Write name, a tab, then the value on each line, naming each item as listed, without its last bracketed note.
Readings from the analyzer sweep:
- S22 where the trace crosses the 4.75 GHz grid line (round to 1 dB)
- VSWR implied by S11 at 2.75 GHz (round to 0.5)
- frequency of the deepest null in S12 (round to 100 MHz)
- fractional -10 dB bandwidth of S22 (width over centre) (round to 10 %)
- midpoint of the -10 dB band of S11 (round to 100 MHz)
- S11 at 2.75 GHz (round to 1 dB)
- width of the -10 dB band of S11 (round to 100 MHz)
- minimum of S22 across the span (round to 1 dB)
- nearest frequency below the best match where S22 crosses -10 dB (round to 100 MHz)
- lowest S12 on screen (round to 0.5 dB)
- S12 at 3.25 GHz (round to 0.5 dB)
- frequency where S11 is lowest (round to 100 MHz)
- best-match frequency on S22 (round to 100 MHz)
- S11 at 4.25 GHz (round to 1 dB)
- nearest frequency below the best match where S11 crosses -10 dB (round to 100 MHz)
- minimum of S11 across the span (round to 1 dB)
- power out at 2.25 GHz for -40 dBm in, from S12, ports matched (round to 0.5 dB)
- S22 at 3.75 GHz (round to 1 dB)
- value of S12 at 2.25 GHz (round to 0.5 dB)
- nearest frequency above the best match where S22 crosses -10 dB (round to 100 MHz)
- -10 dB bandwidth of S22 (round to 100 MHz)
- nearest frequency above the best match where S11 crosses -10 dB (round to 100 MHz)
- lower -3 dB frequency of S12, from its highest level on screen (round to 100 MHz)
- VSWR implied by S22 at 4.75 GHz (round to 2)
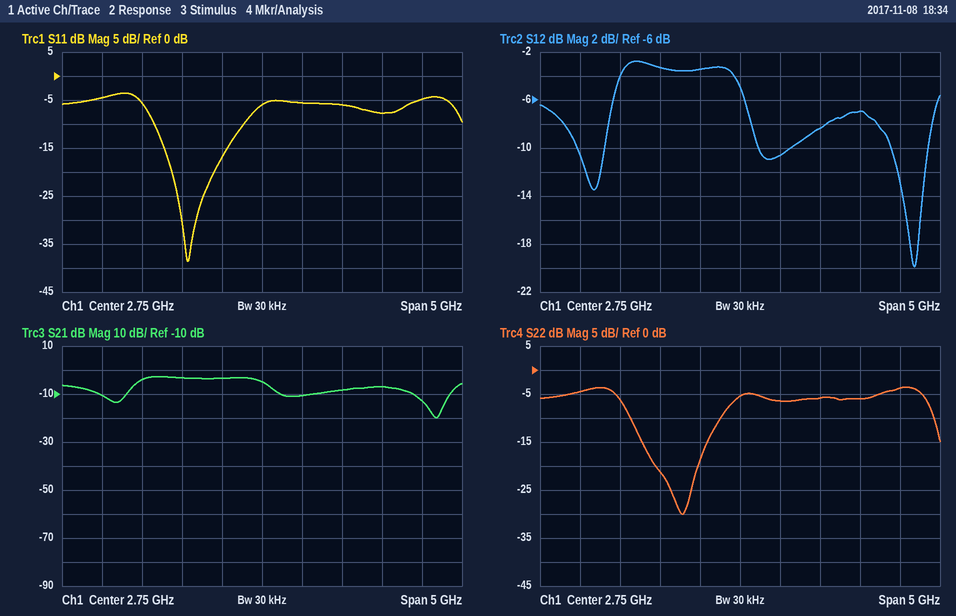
S22 where the trace crosses the 4.75 GHz grid line	-4 dB
VSWR implied by S11 at 2.75 GHz	3.0
frequency of the deepest null in S12	4.9 GHz
fractional -10 dB bandwidth of S22 (width over centre)	60 %
midpoint of the -10 dB band of S11	2.0 GHz
S11 at 2.75 GHz	-6 dB
width of the -10 dB band of S11	1.1 GHz
minimum of S22 across the span	-30 dB
nearest frequency below the best match where S22 crosses -10 dB	1.4 GHz
lowest S12 on screen	-20.0 dB
S12 at 3.25 GHz	-10.5 dB
frequency where S11 is lowest	1.8 GHz
best-match frequency on S22	2.0 GHz
S11 at 4.25 GHz	-8 dB
nearest frequency below the best match where S11 crosses -10 dB	1.4 GHz
minimum of S11 across the span	-39 dB
power out at 2.25 GHz for -40 dBm in, from S12, ports matched	-43.5 dBm
S22 at 3.75 GHz	-6 dB
value of S12 at 2.25 GHz	-3.5 dB
nearest frequency above the best match where S22 crosses -10 dB	2.5 GHz
-10 dB bandwidth of S22	1.1 GHz
nearest frequency above the best match where S11 crosses -10 dB	2.5 GHz
lower -3 dB frequency of S12, from its highest level on screen	1.2 GHz
VSWR implied by S22 at 4.75 GHz	4
